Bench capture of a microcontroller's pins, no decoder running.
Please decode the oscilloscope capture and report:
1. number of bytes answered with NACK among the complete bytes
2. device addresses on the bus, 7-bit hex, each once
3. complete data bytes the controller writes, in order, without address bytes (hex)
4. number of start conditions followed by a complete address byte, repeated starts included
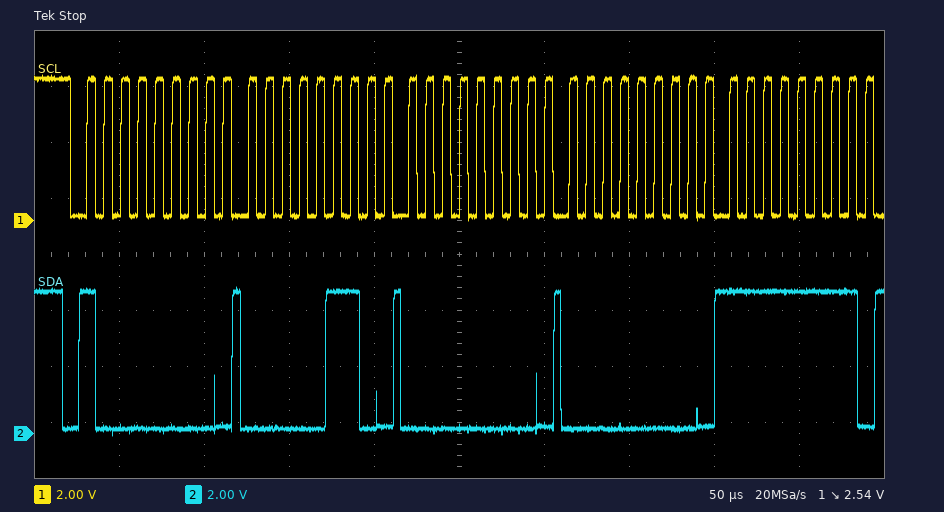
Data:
0
0x40
06 00 00 FF
1
